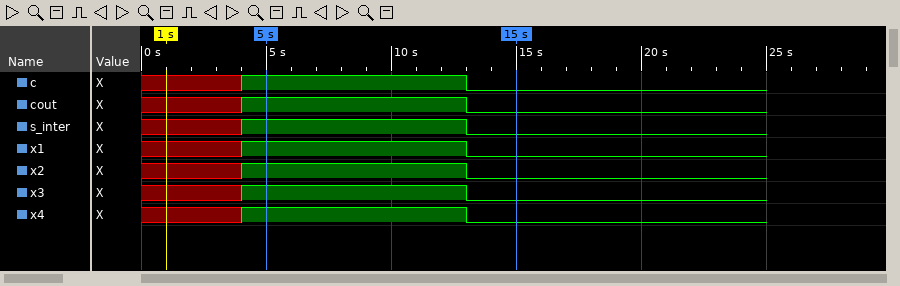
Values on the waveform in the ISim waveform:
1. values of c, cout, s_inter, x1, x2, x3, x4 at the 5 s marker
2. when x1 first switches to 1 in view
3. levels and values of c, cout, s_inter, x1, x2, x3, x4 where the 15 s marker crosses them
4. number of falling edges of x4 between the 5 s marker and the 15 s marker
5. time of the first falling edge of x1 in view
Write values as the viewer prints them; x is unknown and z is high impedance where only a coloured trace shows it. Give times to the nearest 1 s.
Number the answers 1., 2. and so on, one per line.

1. c=1, cout=1, s_inter=1, x1=1, x2=1, x3=1, x4=1
2. 4 s
3. c=0, cout=0, s_inter=0, x1=0, x2=0, x3=0, x4=0
4. 1
5. 13 s
